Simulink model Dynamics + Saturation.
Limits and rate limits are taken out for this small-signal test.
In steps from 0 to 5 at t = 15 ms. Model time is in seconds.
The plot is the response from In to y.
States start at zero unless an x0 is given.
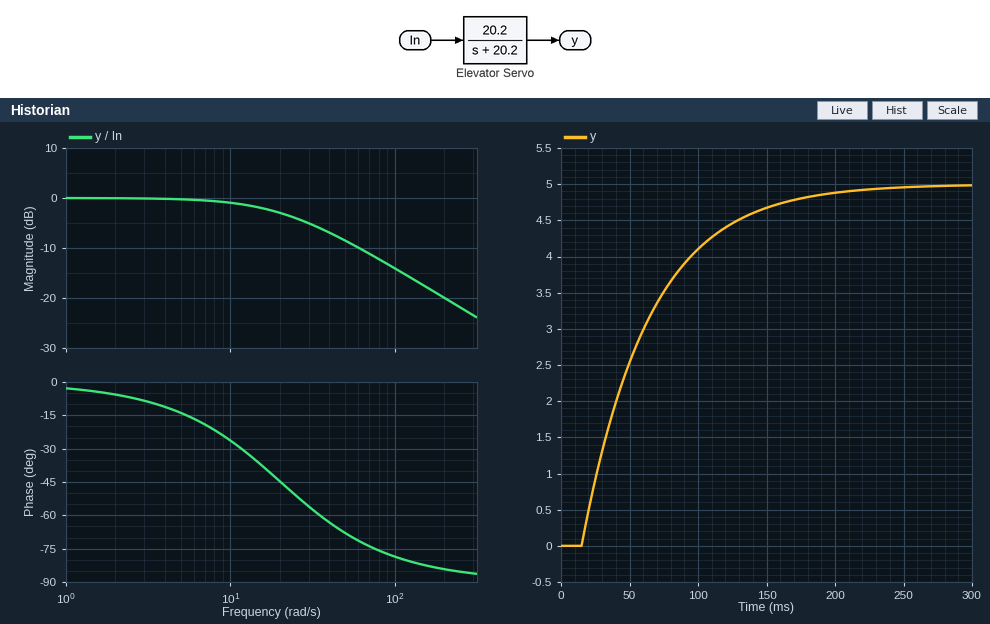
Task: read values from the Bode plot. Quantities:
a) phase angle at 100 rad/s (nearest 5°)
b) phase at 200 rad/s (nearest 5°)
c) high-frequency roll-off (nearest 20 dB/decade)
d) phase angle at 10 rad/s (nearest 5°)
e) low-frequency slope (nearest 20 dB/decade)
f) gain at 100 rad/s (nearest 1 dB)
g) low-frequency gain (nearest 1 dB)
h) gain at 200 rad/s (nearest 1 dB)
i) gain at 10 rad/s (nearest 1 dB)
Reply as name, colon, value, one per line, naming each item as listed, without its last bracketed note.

phase angle at 100 rad/s: -80°
phase at 200 rad/s: -85°
high-frequency roll-off: -20 dB/decade
phase angle at 10 rad/s: -25°
low-frequency slope: 0 dB/decade
gain at 100 rad/s: -14 dB
low-frequency gain: 0 dB
gain at 200 rad/s: -20 dB
gain at 10 rad/s: -1 dB
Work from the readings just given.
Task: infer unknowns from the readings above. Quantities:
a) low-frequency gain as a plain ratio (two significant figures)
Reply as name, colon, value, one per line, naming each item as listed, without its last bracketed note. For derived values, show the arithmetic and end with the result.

low-frequency gain as a plain ratio: 10^(0 / 20) = 1.0
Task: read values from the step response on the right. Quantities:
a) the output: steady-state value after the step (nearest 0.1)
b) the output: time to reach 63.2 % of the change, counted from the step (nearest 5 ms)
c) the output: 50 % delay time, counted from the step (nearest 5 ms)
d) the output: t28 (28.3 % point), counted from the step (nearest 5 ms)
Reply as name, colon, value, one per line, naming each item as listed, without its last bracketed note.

the output: steady-state value after the step: 5.0
the output: time to reach 63.2 % of the change, counted from the step: 50 ms
the output: 50 % delay time, counted from the step: 35 ms
the output: t28 (28.3 % point), counted from the step: 15 ms
